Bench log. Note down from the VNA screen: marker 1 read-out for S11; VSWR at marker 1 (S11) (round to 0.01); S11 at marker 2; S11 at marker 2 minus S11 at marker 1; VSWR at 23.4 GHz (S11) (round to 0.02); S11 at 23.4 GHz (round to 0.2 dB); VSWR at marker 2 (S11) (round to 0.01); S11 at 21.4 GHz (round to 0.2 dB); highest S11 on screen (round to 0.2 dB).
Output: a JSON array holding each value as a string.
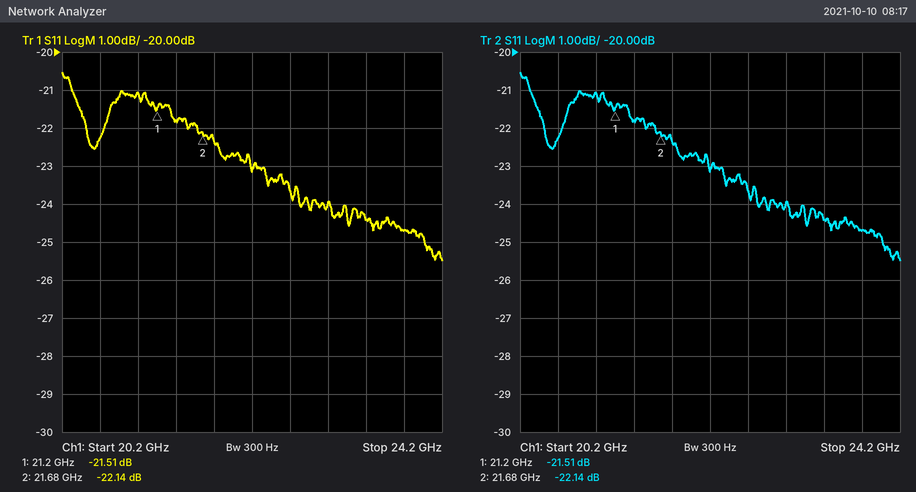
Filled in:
["-21.51 dB", "1.18", "-22.14 dB", "-0.63 dB", "1.12", "-24.4 dB", "1.17", "-21.8 dB", "-20.6 dB"]
